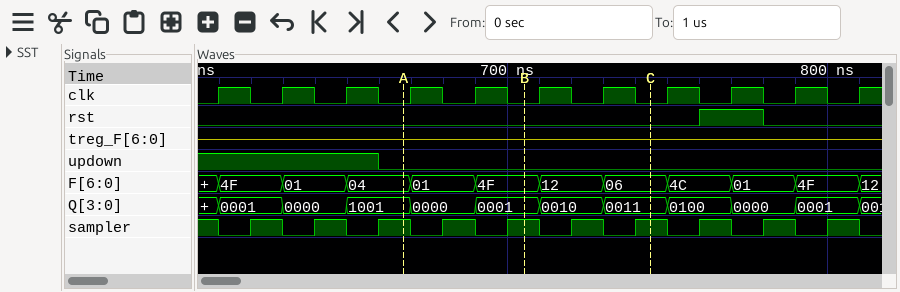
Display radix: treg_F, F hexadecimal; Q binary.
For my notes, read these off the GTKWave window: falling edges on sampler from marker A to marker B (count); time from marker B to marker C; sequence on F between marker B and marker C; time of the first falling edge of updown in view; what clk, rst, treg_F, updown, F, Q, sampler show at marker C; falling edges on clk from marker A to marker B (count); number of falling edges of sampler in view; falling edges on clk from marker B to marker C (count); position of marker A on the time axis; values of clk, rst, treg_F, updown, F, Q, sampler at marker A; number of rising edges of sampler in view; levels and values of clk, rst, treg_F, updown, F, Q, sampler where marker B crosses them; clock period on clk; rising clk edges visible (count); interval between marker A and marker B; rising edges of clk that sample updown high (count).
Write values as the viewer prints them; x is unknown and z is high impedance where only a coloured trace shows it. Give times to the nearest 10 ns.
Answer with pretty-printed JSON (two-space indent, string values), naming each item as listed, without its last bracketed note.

{
  "falling edges on sampler from marker A to marker B": "2",
  "time from marker B to marker C": "40 ns",
  "sequence on F between marker B and marker C": "4F, 12, 06",
  "time of the first falling edge of updown in view": "660 ns",
  "what clk, rst, treg_F, updown, F, Q, sampler show at marker C": "clk=0, rst=0, treg_F=z, updown=0, F=06, Q=0011, sampler=1",
  "falling edges on clk from marker A to marker B": "2",
  "number of falling edges of sampler in view": "11",
  "falling edges on clk from marker B to marker C": "2",
  "position of marker A on the time axis": "670 ns",
  "values of clk, rst, treg_F, updown, F, Q, sampler at marker A": "clk=0, rst=0, treg_F=z, updown=0, F=04, Q=1001, sampler=1",
  "number of rising edges of sampler in view": "10",
  "levels and values of clk, rst, treg_F, updown, F, Q, sampler where marker B crosses them": "clk=0, rst=0, treg_F=z, updown=0, F=4F, Q=0001, sampler=1",
  "clock period on clk": "20 ns",
  "rising clk edges visible": "11",
  "interval between marker A and marker B": "40 ns",
  "rising edges of clk that sample updown high": "3"
}
